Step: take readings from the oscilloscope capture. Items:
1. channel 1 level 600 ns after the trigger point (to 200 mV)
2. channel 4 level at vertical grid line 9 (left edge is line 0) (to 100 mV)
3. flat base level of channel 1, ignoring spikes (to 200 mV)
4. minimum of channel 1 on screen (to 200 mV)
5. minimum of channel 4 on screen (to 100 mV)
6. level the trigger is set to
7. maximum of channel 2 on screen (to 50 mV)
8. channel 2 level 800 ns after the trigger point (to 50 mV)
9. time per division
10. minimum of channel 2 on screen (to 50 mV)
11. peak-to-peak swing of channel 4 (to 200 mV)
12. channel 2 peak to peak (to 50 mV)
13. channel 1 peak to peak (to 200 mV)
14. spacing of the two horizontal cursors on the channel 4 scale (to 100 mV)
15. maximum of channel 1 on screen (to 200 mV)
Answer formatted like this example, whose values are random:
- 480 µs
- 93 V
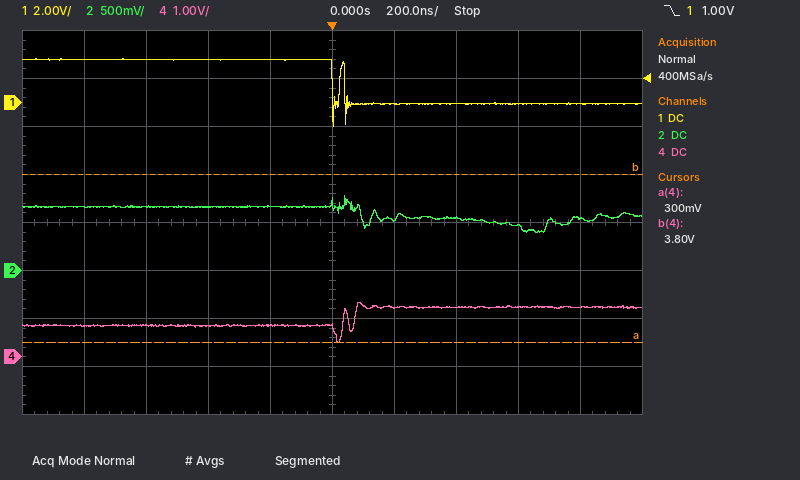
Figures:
- 0.0 V
- 1.0 V
- 0.0 V
- -1.0 V
- 300 mV
- 1.00 V
- 800 mV
- 550 mV
- 200 ns
- 400 mV
- 800 mV
- 400 mV
- 2.8 V
- 3.5 V
- 1.8 V
